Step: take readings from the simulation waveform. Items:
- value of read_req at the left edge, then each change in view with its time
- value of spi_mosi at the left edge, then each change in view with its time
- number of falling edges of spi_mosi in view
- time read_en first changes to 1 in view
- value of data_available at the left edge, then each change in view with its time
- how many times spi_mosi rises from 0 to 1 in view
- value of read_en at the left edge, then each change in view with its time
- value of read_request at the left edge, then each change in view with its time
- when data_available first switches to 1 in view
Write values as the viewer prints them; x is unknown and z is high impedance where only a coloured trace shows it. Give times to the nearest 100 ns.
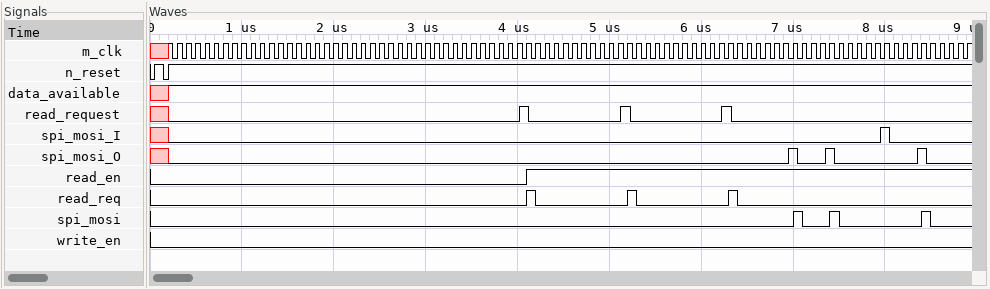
0, 1 at 4100 ns, 0 at 4200 ns, 1 at 5200 ns, 0 at 5300 ns, 1 at 6300 ns, 0 at 6400 ns
0, 1 at 7000 ns, 0 at 7100 ns, 1 at 7400 ns, 0 at 7500 ns, 1 at 8400 ns, 0 at 8500 ns
3
4100 ns
x, 1 at 200 ns
3
0, 1 at 4100 ns
x, 0 at 200 ns, 1 at 4000 ns, 0 at 4100 ns, 1 at 5100 ns, 0 at 5200 ns, 1 at 6200 ns, 0 at 6300 ns
200 ns
